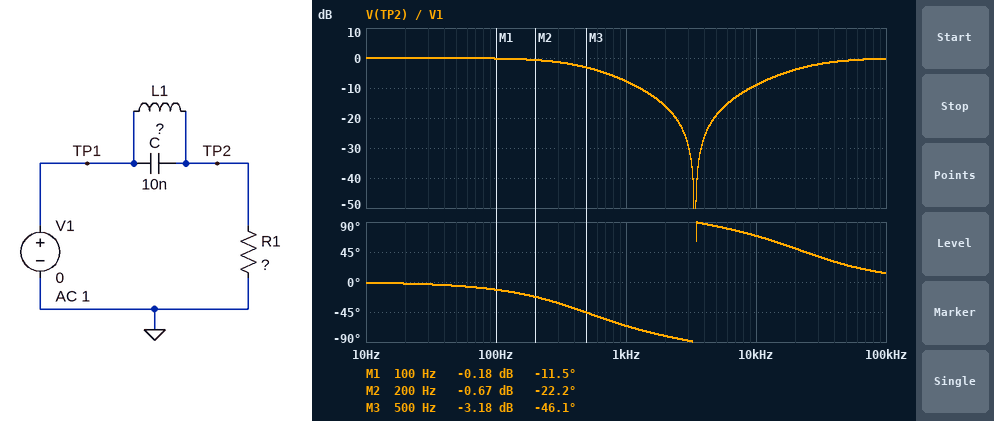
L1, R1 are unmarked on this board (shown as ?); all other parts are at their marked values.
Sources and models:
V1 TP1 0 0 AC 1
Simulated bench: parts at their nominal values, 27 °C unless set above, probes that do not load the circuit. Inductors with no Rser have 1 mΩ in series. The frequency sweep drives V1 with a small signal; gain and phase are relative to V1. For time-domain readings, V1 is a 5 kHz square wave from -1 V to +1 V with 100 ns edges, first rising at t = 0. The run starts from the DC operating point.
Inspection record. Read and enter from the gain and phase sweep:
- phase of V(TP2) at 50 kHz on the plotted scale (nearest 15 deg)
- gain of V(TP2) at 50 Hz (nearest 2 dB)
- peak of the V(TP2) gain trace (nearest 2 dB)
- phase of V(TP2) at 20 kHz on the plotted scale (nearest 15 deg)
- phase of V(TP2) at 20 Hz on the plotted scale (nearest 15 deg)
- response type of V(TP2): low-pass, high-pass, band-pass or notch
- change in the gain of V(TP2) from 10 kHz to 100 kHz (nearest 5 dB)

30 deg
0 dB
0 dB
45 deg
0 deg
notch
10 dB
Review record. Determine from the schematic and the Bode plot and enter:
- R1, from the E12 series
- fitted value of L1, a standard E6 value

680 Ω
220 mH
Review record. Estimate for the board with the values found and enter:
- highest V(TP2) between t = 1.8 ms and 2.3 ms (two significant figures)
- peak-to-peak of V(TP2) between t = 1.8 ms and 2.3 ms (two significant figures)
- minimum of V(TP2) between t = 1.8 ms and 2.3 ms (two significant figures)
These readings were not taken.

1.9 V
3.7 V
-1.9 V
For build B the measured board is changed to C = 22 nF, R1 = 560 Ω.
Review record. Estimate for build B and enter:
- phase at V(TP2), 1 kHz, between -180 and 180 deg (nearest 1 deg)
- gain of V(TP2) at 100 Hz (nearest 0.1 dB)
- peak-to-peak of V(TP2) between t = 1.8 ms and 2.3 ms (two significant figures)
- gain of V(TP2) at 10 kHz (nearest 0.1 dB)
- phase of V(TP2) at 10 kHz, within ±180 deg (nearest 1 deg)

-72 deg
-0.3 dB
3.8 V
-4.6 dB
54 deg
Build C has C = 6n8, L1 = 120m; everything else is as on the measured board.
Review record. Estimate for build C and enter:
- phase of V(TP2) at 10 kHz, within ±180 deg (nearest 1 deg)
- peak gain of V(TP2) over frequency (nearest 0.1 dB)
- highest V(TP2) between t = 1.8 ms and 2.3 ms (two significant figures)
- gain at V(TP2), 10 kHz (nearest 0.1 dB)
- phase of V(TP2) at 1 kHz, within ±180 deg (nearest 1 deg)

79 deg
0 dB
1.7 V
-14.1 dB
-49 deg
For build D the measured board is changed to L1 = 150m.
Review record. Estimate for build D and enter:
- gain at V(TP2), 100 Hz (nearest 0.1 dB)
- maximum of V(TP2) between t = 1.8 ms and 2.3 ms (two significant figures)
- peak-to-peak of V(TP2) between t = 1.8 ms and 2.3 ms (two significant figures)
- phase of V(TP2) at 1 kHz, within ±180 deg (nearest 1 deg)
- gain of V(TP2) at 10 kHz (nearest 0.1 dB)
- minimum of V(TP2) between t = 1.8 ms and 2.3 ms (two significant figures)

-0.1 dB
1.8 V
3.6 V
-56 deg
-9.5 dB
-1.8 V
